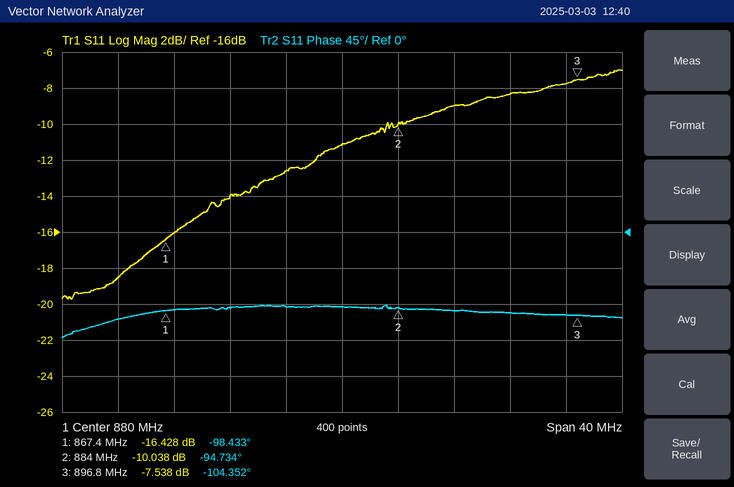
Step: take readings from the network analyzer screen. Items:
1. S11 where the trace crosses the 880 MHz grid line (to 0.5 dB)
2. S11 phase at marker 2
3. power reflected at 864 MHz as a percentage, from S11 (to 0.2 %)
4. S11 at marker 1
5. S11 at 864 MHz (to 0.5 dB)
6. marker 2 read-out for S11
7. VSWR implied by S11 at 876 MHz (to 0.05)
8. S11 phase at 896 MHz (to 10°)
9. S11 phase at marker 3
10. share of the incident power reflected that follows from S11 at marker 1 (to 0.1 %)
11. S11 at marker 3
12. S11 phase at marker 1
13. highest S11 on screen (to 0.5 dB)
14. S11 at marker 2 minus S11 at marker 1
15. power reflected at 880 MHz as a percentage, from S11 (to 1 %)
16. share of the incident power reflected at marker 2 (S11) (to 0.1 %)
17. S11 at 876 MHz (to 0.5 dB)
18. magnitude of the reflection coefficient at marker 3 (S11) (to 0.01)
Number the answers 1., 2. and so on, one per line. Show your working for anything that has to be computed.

1. -11.0 dB
2. -94.734°
3. 10^(-18.5/10) ≈ 1.4 %
4. -16.428 dB
5. -18.5 dB
6. -10.038 dB
7. |Γ| = 10^(-12.5/20) = 0.2371; VSWR = (1 + 0.2371)/(1 − 0.2371) ≈ 1.62, so 1.60 to the nearest 0.05
8. -100°
9. -104.352°
10. 10^(-16.428/10) ≈ 2.3 %
11. -7.538 dB
12. -98.433°
13. -7.0 dB
14. -10.038 − (-16.428) = 6.390 dB
15. 10^(-11/10) ≈ 8 %
16. 10^(-10.038/10) ≈ 9.9 %
17. -12.5 dB
18. 10^(-7.538/20) ≈ 0.42
